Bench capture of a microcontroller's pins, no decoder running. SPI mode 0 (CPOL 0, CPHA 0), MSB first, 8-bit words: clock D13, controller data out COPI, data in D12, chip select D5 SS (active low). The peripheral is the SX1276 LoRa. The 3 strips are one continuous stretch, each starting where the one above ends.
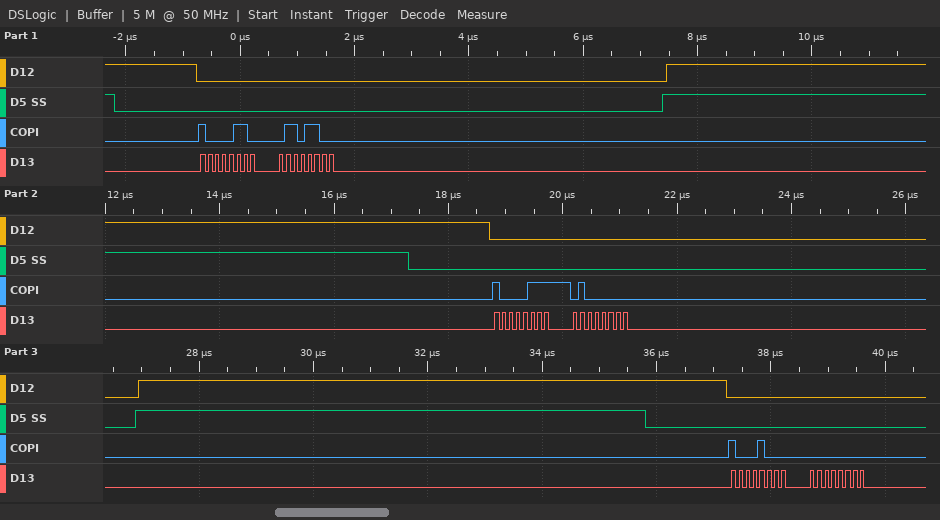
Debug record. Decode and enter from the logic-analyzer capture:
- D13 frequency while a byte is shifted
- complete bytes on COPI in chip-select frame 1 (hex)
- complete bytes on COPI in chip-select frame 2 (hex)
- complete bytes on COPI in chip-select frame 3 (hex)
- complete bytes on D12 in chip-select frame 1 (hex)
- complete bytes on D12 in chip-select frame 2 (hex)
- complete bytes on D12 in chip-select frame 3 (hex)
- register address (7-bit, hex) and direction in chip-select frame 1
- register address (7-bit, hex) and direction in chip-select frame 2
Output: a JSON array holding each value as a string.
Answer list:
["8 MHz", "0x86 0x6C", "0x87 0x40", "0x88 0x00", "0x00 0x00", "0x00 0x00", "0x00 0x00", "0x06 write", "0x07 write"]
